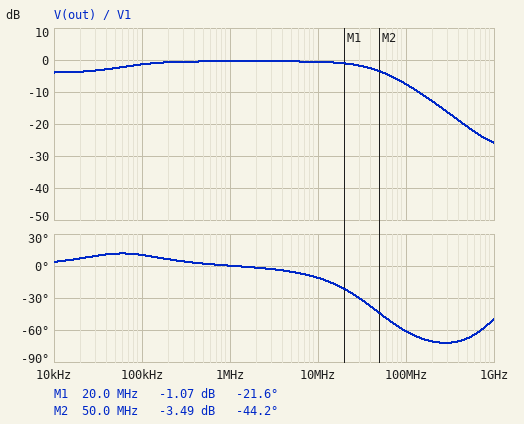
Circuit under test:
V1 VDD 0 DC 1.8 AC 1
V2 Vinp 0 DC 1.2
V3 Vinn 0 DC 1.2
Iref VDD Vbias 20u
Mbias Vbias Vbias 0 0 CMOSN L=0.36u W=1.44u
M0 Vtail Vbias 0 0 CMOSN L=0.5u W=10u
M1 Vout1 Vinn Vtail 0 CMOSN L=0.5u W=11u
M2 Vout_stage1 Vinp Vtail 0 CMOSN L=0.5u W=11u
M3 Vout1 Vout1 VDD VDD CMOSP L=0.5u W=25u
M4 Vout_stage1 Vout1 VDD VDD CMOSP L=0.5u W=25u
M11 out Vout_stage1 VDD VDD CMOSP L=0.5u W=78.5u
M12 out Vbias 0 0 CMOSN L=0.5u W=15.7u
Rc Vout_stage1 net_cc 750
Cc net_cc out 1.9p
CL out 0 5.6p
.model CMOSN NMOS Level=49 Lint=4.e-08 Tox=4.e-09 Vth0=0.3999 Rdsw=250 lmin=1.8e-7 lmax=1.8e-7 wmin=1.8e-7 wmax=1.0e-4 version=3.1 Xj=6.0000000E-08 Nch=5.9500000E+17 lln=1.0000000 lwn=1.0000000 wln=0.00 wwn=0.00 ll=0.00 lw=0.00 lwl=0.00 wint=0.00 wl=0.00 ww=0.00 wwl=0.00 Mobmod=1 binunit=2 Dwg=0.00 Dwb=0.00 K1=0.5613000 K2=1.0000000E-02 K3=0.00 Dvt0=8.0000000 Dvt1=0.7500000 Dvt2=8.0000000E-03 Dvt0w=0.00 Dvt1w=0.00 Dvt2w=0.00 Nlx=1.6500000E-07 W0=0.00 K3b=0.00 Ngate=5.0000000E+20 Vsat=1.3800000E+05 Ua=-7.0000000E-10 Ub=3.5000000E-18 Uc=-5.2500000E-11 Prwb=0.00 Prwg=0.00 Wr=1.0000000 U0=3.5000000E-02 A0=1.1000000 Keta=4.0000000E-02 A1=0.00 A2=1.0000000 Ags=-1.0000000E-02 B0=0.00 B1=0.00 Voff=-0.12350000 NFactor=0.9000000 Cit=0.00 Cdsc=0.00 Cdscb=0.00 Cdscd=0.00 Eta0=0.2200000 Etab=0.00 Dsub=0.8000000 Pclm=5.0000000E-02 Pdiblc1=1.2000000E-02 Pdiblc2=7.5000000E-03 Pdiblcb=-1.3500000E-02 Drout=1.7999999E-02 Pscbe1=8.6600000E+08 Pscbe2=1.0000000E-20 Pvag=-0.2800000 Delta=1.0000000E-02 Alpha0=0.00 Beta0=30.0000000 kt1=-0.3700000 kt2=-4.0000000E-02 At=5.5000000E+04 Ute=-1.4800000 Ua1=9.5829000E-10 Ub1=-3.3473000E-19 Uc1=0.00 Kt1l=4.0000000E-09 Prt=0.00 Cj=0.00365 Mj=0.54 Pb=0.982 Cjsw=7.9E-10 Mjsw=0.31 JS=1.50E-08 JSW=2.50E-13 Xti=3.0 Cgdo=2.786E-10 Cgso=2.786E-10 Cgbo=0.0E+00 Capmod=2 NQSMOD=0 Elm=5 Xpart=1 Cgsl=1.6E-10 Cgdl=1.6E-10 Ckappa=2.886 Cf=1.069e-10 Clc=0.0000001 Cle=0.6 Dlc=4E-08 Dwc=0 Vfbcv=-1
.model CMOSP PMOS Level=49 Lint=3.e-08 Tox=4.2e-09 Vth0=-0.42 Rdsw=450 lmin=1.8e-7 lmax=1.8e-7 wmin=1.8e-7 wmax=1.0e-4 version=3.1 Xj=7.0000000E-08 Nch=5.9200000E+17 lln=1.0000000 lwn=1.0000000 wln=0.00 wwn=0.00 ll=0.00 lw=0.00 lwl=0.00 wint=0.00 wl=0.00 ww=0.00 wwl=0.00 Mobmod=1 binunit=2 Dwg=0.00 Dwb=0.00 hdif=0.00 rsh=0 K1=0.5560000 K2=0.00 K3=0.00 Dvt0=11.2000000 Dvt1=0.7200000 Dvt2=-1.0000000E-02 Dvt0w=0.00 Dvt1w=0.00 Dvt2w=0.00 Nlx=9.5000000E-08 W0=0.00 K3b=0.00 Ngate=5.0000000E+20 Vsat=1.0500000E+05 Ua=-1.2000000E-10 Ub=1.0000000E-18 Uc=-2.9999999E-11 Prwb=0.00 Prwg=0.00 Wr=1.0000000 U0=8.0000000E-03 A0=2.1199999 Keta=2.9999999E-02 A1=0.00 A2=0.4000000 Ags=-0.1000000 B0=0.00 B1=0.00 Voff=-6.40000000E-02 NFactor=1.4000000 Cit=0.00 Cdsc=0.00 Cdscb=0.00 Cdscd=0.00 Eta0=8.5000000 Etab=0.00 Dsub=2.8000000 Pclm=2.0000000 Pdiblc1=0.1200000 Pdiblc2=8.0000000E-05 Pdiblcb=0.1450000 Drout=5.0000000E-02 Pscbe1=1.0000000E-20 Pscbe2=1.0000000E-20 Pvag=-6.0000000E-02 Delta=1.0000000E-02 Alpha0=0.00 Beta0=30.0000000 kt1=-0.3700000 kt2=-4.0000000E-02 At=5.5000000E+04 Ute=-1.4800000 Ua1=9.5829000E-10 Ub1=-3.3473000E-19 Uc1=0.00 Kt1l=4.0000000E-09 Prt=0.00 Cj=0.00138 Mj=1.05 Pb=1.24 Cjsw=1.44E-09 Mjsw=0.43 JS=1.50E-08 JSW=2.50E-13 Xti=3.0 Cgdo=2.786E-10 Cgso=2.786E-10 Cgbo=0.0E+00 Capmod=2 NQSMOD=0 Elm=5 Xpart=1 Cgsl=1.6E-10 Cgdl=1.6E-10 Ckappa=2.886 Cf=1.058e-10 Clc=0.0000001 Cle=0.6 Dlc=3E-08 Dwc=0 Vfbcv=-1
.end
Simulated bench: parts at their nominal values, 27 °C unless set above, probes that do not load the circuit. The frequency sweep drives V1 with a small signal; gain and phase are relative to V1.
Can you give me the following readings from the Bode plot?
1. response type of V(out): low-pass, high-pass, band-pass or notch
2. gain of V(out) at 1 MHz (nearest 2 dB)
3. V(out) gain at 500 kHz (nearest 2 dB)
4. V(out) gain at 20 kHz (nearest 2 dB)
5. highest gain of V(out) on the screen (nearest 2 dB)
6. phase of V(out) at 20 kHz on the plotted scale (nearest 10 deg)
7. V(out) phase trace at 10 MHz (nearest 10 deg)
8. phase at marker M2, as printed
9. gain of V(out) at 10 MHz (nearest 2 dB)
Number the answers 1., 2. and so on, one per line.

1. low-pass
2. 0 dB
3. 0 dB
4. -4 dB
5. 0 dB
6. 10 deg
7. -10 deg
8. -44.2 deg
9. 0 dB
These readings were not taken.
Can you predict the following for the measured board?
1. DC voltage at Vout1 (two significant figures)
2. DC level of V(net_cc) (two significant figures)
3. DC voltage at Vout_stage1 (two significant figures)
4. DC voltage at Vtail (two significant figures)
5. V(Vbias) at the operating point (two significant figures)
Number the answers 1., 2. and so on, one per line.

1. 1.1 V
2. 1.1 V
3. 1.1 V
4. 460 mV
5. 690 mV
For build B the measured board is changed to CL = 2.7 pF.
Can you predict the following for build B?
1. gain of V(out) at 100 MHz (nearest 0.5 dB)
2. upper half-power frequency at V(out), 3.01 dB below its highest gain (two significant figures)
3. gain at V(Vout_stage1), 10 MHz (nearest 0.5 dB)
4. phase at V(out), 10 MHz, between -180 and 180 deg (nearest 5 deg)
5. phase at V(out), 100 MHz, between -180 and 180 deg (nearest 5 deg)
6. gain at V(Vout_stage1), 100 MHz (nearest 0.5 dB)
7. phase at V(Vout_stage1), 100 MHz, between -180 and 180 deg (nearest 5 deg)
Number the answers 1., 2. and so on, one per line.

1. -3.5 dB
2. 96 MHz
3. 0 dB
4. -5 deg
5. -45 deg
6. -4.0 dB
7. -30 deg
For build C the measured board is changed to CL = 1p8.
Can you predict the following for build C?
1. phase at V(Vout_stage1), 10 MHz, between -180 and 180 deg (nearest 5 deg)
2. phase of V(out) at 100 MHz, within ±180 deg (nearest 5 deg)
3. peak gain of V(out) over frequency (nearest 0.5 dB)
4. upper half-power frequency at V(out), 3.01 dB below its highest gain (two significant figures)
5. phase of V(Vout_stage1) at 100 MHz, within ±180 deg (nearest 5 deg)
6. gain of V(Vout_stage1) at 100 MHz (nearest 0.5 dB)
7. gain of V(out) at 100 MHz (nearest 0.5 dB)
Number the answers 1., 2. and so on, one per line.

1. -5 deg
2. -35 deg
3. 0 dB
4. 140 MHz
5. -25 deg
6. -2.5 dB
7. -2.0 dB
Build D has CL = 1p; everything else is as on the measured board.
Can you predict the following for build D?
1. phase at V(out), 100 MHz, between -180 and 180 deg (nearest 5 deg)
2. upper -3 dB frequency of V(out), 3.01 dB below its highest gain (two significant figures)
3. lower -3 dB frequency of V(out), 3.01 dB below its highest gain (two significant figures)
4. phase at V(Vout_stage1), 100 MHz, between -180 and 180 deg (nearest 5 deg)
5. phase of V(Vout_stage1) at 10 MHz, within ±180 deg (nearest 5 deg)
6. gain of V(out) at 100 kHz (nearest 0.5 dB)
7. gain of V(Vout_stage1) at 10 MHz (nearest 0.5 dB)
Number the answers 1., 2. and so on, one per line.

1. -20 deg
2. 230 MHz
3. 32 kHz
4. -15 deg
5. 0 deg
6. -1.0 dB
7. 0 dB
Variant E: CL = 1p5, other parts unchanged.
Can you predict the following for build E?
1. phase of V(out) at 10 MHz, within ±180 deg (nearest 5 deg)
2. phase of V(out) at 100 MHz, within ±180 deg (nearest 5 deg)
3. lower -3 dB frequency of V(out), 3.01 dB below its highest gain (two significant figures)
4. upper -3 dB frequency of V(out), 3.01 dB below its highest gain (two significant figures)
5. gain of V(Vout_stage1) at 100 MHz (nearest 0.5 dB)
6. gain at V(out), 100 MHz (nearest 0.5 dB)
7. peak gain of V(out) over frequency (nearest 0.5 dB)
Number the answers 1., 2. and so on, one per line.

1. -5 deg
2. -30 deg
3. 31 kHz
4. 160 MHz
5. -2.0 dB
6. -1.5 dB
7. 0 dB
